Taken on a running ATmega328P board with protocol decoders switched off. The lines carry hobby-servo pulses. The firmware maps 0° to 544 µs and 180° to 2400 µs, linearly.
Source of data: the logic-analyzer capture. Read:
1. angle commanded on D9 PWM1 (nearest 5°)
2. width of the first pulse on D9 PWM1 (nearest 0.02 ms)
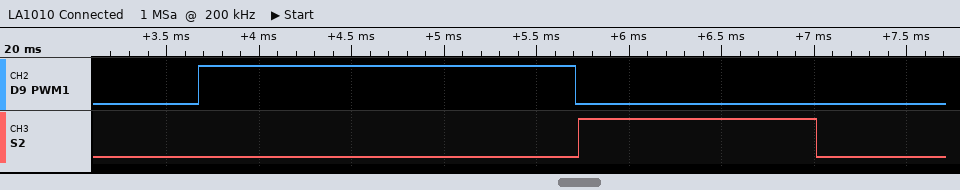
145°
2.04 ms
